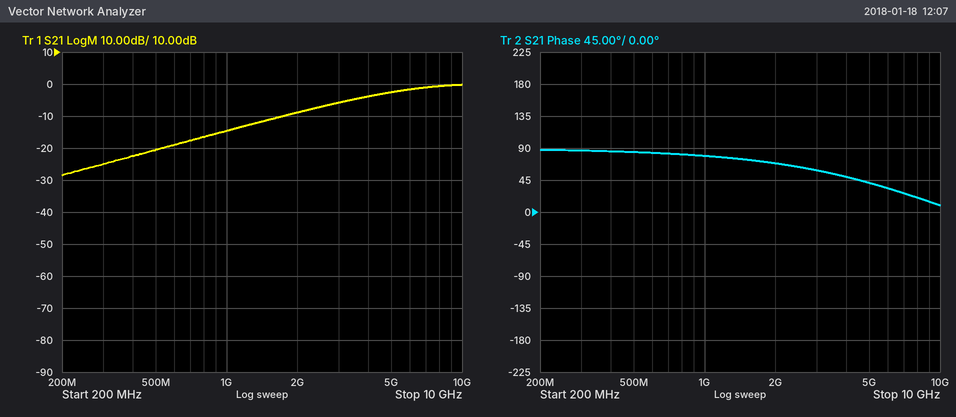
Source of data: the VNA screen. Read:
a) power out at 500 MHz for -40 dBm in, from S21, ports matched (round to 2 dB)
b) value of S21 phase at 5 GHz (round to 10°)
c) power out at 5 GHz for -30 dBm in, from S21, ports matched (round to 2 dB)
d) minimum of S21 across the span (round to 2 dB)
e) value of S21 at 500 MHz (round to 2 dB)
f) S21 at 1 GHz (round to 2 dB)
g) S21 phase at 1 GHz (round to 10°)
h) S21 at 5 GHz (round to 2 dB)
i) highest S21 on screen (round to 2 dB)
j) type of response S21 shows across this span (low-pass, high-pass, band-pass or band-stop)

-60 dBm
40°
-32 dBm
-28 dB
-20 dB
-14 dB
80°
-2 dB
0 dB
high-pass
